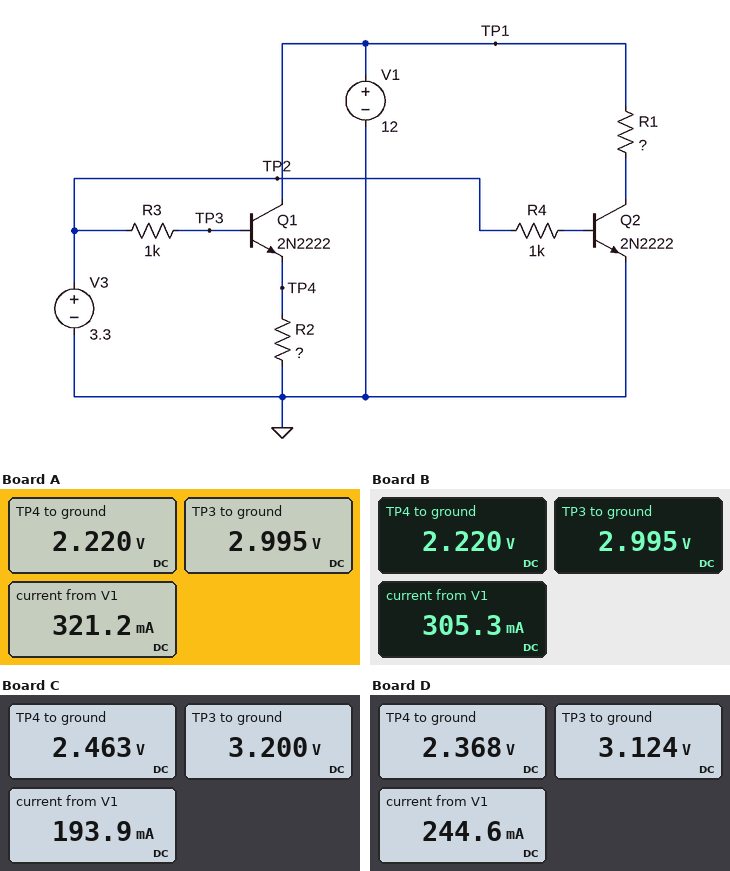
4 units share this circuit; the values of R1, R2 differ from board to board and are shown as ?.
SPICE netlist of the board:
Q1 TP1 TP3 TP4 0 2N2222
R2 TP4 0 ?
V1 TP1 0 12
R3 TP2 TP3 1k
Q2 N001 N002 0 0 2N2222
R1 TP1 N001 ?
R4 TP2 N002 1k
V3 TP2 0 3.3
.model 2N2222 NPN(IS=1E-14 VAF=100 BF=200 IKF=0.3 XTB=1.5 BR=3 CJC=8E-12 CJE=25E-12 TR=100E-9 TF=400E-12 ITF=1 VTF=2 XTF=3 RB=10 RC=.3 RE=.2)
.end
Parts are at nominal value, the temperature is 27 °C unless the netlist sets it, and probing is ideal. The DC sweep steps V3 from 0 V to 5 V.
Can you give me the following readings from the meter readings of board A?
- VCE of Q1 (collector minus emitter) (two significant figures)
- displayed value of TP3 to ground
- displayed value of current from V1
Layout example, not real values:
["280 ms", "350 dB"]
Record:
["9.8 V", "2.995 V", "321.2 mA"]
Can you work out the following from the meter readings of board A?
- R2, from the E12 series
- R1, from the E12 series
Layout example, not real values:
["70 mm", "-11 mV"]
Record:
["39 Ω", "33 Ω"]
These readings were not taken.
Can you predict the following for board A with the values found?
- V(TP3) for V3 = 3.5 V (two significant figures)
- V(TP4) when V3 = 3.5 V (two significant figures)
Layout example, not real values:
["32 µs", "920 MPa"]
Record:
["3.2 V", "2.4 V"]
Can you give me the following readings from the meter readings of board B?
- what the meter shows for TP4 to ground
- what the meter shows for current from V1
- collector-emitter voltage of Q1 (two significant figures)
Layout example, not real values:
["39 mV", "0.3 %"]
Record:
["2.220 V", "305.3 mA", "9.8 V"]
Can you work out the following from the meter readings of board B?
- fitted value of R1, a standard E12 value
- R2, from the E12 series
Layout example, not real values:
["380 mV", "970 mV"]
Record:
["47 Ω", "39 Ω"]
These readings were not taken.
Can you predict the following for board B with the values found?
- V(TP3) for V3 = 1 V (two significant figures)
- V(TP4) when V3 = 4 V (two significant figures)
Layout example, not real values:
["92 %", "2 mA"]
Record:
["970 mV", "2.8 V"]
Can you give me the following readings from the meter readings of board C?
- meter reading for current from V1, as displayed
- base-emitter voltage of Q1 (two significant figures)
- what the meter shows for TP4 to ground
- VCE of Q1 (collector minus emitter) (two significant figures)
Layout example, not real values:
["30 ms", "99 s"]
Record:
["193.9 mA", "740 mV", "2.463 V", "9.5 V"]
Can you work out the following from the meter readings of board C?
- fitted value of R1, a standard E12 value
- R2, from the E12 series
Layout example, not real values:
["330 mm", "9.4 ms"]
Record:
["68 Ω", "120 Ω"]
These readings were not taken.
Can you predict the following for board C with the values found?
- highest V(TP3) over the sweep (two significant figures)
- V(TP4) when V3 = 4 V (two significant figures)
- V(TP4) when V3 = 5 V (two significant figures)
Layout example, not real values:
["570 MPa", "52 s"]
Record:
["4.8 V", "3.1 V", "4.1 V"]
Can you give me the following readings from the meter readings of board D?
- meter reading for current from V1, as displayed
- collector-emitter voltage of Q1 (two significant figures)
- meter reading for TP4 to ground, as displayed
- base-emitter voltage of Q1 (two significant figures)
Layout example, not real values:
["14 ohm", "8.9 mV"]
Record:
["244.6 mA", "9.6 V", "2.368 V", "760 mV"]
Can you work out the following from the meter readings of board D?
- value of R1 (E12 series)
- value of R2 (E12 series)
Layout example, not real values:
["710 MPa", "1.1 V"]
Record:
["56 Ω", "68 Ω"]
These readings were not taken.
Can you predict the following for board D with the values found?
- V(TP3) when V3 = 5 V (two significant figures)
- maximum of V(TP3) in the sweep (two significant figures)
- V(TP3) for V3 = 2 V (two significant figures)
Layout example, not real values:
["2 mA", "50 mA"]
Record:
["4.7 V", "4.7 V", "1.9 V"]
